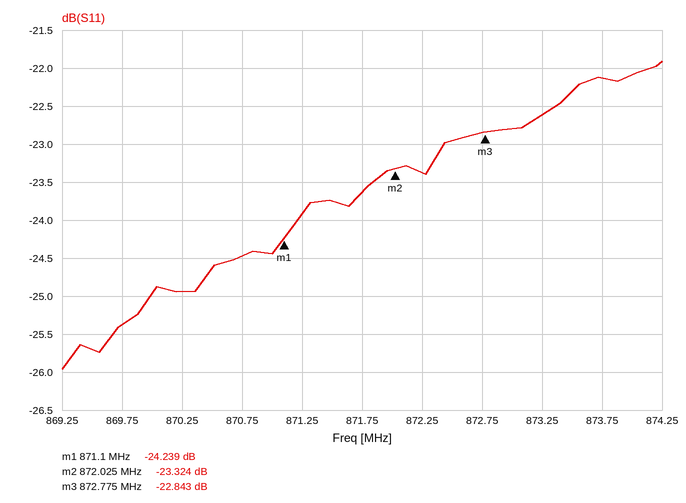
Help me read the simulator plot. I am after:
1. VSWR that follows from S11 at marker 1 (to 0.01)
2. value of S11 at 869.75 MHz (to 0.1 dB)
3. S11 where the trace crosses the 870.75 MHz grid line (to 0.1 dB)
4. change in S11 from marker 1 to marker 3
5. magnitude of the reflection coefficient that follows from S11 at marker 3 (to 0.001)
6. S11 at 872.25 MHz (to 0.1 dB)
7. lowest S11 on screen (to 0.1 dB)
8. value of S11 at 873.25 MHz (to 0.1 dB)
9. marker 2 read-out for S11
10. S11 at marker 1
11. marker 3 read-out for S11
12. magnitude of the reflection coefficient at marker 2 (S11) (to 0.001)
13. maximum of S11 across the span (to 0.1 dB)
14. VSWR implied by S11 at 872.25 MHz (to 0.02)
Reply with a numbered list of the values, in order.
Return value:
1. 1.13
2. -25.4 dB
3. -24.5 dB
4. 1.396 dB
5. 0.072
6. -23.4 dB
7. -26.0 dB
8. -22.6 dB
9. -23.324 dB
10. -24.239 dB
11. -22.843 dB
12. 0.068
13. -21.9 dB
14. 1.14
